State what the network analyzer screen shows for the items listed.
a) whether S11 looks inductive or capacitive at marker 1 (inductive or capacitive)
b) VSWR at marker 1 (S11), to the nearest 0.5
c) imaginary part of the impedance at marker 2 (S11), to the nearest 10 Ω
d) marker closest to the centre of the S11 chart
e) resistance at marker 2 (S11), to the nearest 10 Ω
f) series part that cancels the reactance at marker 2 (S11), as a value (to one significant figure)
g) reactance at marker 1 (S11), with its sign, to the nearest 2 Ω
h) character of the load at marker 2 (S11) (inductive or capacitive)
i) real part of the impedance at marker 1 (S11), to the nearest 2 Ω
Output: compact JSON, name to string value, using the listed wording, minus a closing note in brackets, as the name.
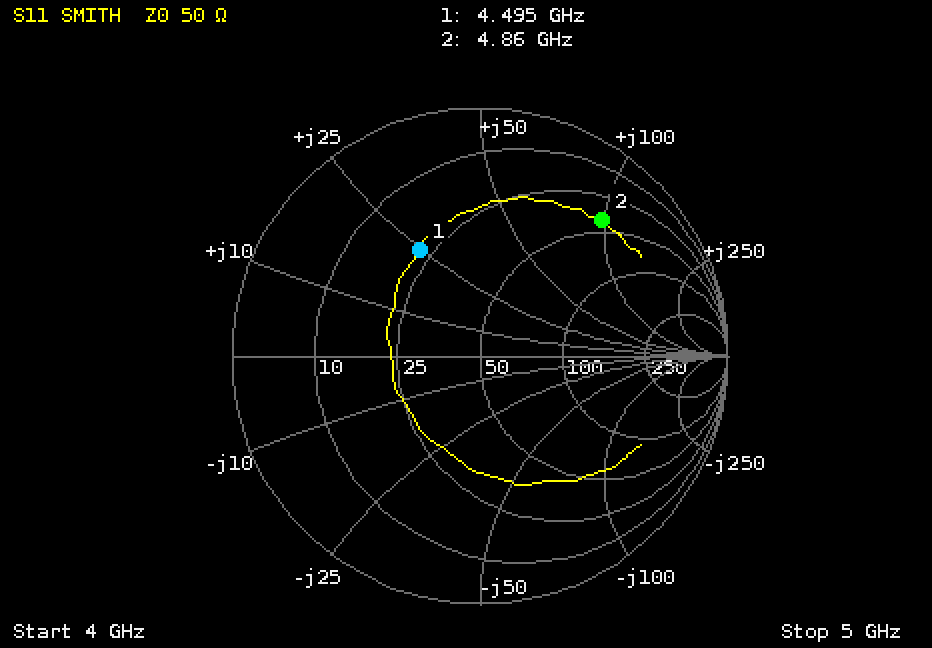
{"whether S11 looks inductive or capacitive at marker 1": "inductive", "VSWR at marker 1 (S11), to the nearest 0.5": "3.0", "imaginary part of the impedance at marker 2 (S11), to the nearest 10 Ω": "+100 Ω", "marker closest to the centre of the S11 chart": "marker 1", "resistance at marker 2 (S11), to the nearest 10 Ω": "40 Ω", "series part that cancels the reactance at marker 2 (S11), as a value": "300 fF", "reactance at marker 1 (S11), with its sign, to the nearest 2 Ω": "+24 Ω", "character of the load at marker 2 (S11)": "inductive", "real part of the impedance at marker 1 (S11), to the nearest 2 Ω": "22 Ω"}
